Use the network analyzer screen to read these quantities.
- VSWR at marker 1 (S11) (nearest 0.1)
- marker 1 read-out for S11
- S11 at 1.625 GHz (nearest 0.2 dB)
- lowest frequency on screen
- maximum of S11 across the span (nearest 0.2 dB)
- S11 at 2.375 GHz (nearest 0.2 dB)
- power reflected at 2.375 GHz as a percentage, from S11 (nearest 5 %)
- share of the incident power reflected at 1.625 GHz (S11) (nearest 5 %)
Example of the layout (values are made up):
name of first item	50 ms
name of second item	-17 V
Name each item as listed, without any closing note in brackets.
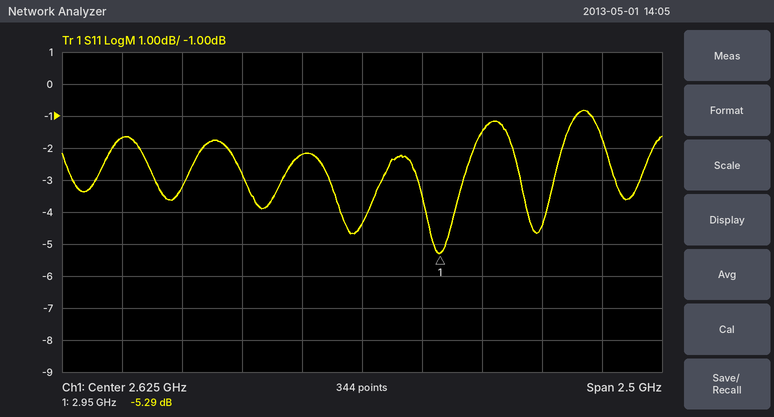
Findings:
VSWR at marker 1 (S11)	3.4
marker 1 read-out for S11	-5.29 dB
S11 at 1.625 GHz	-1.6 dB
lowest frequency on screen	1.375 GHz
maximum of S11 across the span	-0.8 dB
S11 at 2.375 GHz	-2.2 dB
power reflected at 2.375 GHz as a percentage, from S11	60 %
share of the incident power reflected at 1.625 GHz (S11)	70 %
